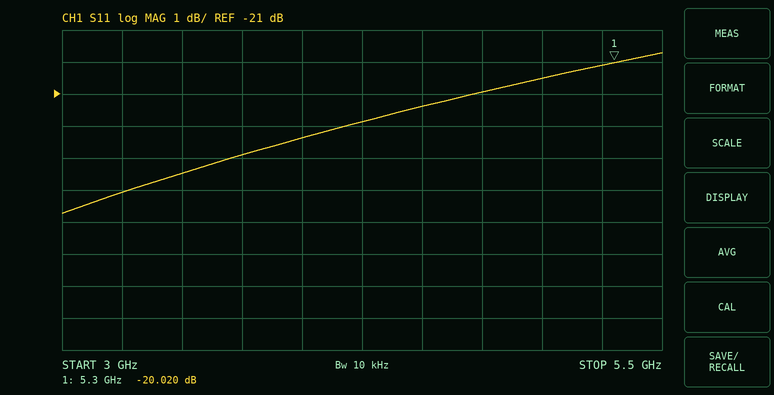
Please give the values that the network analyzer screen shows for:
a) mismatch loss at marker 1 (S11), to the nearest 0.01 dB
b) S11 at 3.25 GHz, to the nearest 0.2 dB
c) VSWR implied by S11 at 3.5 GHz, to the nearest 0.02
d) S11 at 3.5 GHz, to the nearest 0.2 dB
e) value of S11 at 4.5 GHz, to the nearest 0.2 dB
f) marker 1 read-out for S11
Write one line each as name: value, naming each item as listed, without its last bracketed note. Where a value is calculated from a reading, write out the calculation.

mismatch loss at marker 1 (S11), to the nearest 0.01 dB: −10 log10(1 − 10^(-20.02/10)) ≈ 0.04 dB
S11 at 3.25 GHz, to the nearest 0.2 dB: -24.0 dB
VSWR implied by S11 at 3.5 GHz, to the nearest 0.02: |Γ| = 10^(-23.4/20) = 0.0676; VSWR = (1 + 0.0676)/(1 − 0.0676) ≈ 1.15, so 1.14 to the nearest 0.02
S11 at 3.5 GHz, to the nearest 0.2 dB: -23.4 dB
value of S11 at 4.5 GHz, to the nearest 0.2 dB: -21.4 dB
marker 1 read-out for S11: -20.020 dB
